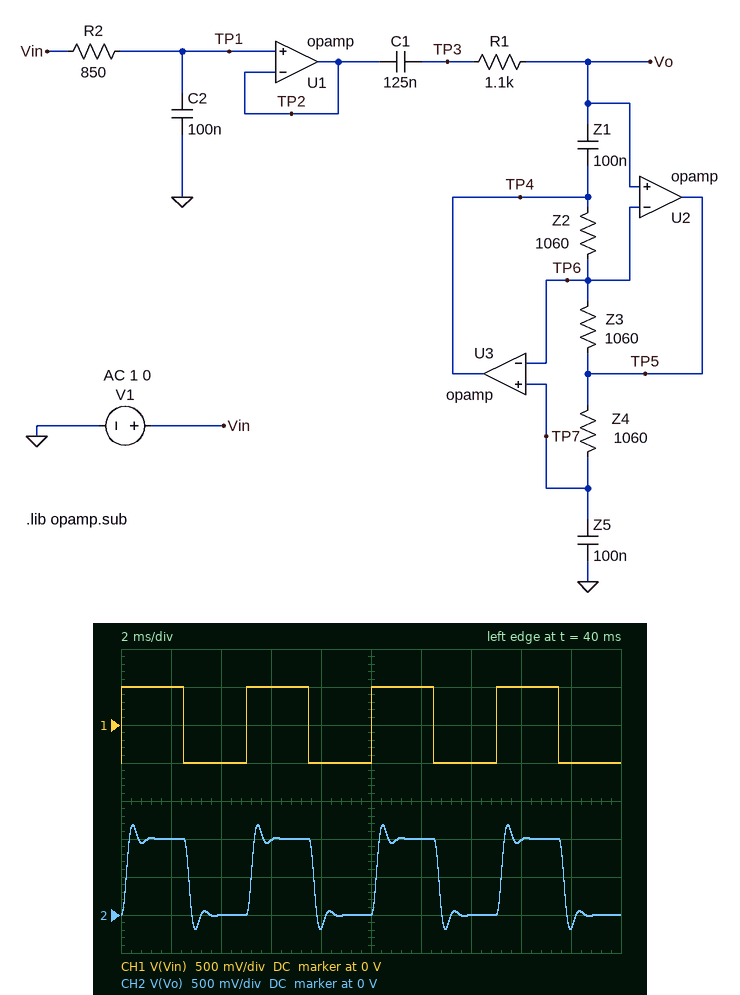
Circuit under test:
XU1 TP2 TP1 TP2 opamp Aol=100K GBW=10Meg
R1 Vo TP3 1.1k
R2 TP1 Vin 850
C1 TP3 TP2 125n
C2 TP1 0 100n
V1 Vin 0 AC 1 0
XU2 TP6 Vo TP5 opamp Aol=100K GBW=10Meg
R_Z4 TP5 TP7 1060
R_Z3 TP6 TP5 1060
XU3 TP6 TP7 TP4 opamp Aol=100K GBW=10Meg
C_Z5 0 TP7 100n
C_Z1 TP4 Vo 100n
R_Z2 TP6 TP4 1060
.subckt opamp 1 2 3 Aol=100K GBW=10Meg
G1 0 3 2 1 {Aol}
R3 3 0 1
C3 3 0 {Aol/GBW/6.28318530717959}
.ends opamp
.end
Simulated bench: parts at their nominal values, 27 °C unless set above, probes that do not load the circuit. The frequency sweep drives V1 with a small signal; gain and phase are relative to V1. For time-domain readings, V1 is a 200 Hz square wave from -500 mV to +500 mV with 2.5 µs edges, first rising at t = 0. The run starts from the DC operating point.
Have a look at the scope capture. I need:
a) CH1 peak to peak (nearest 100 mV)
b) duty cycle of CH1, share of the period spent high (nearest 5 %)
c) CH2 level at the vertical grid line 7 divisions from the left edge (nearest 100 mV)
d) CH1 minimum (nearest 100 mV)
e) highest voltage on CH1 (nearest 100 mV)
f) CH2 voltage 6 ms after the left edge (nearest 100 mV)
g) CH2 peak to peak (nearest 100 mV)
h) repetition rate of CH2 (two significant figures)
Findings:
1.0 V
50 %
0 V
-500 mV
500 mV
1.0 V
1.4 V
200 Hz
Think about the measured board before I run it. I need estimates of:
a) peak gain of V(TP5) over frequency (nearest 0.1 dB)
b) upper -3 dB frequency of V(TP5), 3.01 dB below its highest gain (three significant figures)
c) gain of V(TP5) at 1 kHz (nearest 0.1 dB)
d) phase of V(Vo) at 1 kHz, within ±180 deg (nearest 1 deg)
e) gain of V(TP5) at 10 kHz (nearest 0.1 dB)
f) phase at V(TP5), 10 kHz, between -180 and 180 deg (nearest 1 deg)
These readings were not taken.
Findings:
3.5 dB
1.79 kHz
2.9 dB
-73 deg
-31.3 dB
-171 deg
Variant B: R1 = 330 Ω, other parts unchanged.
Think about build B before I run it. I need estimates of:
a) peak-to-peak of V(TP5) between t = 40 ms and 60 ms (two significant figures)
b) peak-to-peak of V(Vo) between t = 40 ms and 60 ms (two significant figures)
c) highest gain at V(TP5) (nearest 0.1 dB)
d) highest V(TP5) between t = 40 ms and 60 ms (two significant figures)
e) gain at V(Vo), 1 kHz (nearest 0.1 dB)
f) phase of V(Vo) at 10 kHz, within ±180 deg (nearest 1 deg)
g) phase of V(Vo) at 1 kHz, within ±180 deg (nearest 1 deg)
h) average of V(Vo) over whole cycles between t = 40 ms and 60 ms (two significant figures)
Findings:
1.2 V
1.0 V
0.4 dB
1.1 V
-1.2 dB
123 deg
-60 deg
500 mV
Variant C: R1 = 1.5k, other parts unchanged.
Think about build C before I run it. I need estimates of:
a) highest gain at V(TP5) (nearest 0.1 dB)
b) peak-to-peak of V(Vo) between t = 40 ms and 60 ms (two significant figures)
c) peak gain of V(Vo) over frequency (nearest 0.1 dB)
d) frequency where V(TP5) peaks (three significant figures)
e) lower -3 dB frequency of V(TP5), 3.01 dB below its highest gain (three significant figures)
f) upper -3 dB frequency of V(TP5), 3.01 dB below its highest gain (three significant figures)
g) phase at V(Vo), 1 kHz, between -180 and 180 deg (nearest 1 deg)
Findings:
4.6 dB
1.5 V
2.7 dB
1.13 kHz
562 Hz
1.52 kHz
-83 deg
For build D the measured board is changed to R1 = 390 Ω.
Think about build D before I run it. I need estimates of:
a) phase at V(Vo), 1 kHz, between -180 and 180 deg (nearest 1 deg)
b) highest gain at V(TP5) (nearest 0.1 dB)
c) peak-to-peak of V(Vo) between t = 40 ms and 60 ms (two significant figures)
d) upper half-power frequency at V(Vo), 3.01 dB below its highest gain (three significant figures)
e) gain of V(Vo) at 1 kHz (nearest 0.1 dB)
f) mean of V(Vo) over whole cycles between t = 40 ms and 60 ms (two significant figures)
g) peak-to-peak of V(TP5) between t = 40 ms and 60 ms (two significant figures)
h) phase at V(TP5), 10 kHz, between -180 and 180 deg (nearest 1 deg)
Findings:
-61 deg
0.7 dB
1.0 V
1.70 kHz
-1.0 dB
500 mV
1.2 V
-159 deg
